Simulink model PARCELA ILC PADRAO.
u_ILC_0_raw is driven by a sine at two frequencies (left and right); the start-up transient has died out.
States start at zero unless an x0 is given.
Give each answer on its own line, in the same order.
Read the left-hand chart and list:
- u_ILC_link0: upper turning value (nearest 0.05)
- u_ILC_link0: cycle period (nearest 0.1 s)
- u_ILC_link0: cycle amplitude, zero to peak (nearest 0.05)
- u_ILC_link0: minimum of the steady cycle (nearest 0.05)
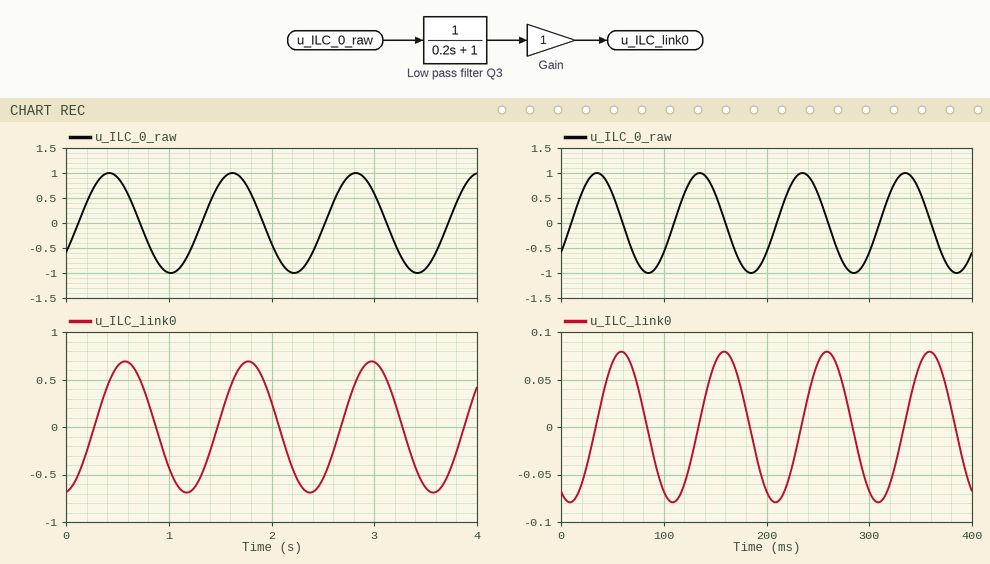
0.70
1.2 s
0.70
-0.70
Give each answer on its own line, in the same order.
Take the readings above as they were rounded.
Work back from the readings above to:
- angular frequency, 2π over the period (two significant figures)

5.2 rad/s
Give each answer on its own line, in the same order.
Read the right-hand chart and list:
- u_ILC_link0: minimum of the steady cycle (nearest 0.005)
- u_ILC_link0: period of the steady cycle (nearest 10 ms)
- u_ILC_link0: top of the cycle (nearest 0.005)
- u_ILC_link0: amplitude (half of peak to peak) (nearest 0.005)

-0.080
100 ms
0.080
0.080
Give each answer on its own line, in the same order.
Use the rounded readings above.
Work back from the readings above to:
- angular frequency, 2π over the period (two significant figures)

0.063 rad/ms
